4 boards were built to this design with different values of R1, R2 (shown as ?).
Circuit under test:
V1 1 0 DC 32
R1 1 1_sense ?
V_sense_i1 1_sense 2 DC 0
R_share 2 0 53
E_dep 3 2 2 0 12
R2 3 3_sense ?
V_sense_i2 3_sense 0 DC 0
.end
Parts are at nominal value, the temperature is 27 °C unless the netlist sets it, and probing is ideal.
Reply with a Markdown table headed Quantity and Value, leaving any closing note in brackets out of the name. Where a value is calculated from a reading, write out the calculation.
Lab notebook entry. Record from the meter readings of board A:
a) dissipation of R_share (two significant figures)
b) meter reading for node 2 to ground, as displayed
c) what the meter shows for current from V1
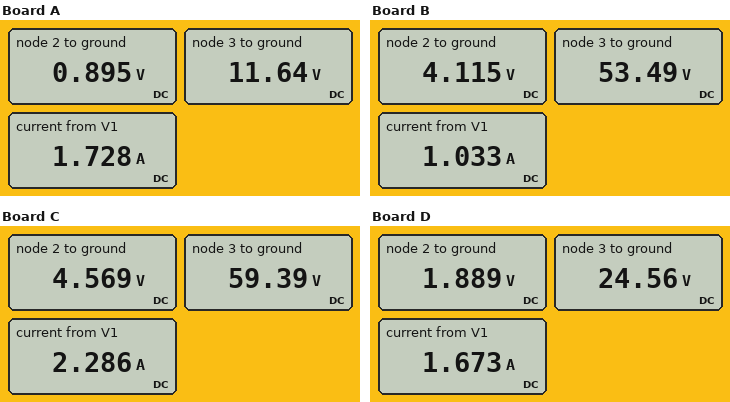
| Quantity | Value |
|---|---|
| dissipation of R_share | (895 mV)^2 / 53 Ω = 15 mW |
| meter reading for node 2 to ground, as displayed | 0.895 V |
| what the meter shows for current from V1 | 1.728 A |
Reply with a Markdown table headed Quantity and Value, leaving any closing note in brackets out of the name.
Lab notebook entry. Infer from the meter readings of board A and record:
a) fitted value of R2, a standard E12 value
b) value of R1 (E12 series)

| Quantity | Value |
|---|---|
| fitted value of R2, a standard E12 value | 6.8 Ω |
| value of R1 | 18 Ω |
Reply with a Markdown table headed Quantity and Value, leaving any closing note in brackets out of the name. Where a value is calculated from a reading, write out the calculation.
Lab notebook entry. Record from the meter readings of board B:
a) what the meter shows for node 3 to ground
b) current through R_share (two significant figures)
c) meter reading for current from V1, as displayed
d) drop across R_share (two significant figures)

| Quantity | Value |
|---|---|
| what the meter shows for node 3 to ground | 53.49 V |
| current through R_share | (4.115 V) / 53 Ω = 78 mA |
| meter reading for current from V1, as displayed | 1.033 A |
| drop across R_share | 4.115 V = 4.1 V |
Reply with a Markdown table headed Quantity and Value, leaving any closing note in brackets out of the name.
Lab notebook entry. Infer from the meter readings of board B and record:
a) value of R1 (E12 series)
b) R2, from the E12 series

| Quantity | Value |
|---|---|
| value of R1 | 27 Ω |
| R2, from the E12 series | 56 Ω |
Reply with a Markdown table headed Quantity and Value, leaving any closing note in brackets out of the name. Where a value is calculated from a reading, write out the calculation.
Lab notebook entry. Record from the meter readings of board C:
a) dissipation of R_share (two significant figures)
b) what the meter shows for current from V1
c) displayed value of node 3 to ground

| Quantity | Value |
|---|---|
| dissipation of R_share | (4.569 V)^2 / 53 Ω = 390 mW |
| what the meter shows for current from V1 | 2.286 A |
| displayed value of node 3 to ground | 59.39 V |
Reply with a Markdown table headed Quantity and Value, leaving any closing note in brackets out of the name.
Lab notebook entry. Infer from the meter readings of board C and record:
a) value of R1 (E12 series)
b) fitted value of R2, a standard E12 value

| Quantity | Value |
|---|---|
| value of R1 | 12 Ω |
| fitted value of R2, a standard E12 value | 27 Ω |
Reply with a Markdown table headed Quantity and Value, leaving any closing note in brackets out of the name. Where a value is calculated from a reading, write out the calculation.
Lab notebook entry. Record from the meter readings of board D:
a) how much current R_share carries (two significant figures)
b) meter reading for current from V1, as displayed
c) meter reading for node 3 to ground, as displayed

| Quantity | Value |
|---|---|
| how much current R_share carries | (1.889 V) / 53 Ω = 36 mA |
| meter reading for current from V1, as displayed | 1.673 A |
| meter reading for node 3 to ground, as displayed | 24.56 V |
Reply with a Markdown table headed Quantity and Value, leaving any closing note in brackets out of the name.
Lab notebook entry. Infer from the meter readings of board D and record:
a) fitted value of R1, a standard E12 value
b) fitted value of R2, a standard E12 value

| Quantity | Value |
|---|---|
| fitted value of R1, a standard E12 value | 18 Ω |
| fitted value of R2, a standard E12 value | 15 Ω |
